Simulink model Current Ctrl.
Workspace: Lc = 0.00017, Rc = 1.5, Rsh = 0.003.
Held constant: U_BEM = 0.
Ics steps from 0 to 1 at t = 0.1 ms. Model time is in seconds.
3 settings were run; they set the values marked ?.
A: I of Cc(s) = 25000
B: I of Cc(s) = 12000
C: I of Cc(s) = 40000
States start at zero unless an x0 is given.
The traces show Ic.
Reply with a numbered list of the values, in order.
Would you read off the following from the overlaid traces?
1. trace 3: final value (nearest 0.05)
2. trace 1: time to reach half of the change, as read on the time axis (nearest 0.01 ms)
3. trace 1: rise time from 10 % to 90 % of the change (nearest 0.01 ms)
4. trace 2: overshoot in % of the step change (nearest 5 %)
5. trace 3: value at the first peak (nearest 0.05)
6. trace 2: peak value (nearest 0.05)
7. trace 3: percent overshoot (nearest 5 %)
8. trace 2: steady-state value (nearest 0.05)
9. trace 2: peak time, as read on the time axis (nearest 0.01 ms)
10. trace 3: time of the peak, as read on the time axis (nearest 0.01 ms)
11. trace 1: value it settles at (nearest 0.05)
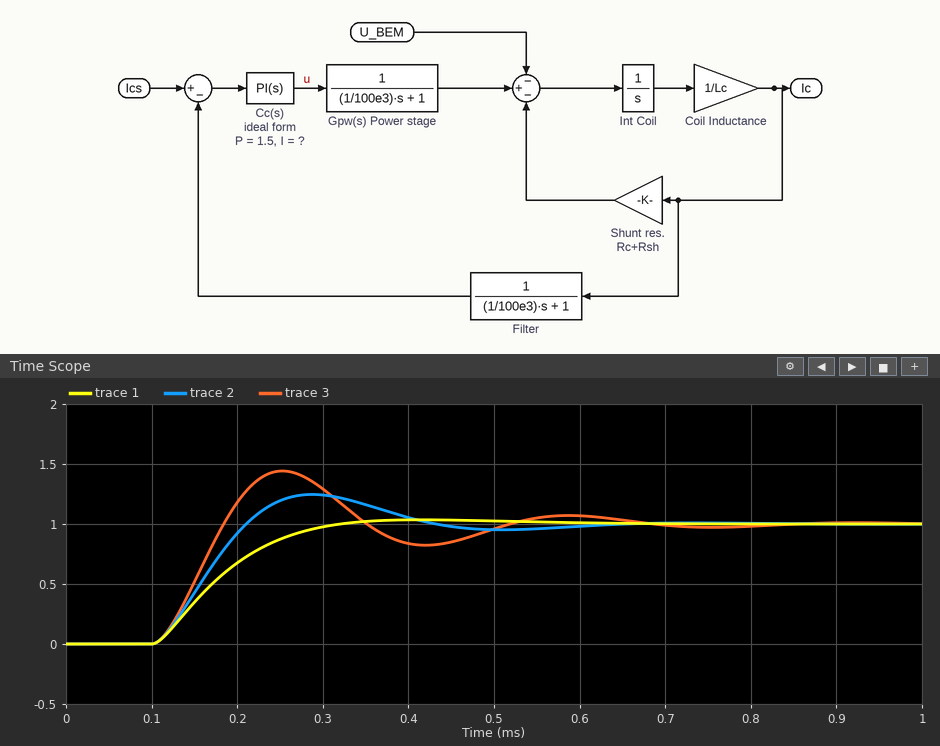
1. 1.00
2. 0.17 ms
3. 0.14 ms
4. 25 %
5. 1.45
6. 1.25
7. 45 %
8. 1.00
9. 0.29 ms
10. 0.25 ms
11. 1.00
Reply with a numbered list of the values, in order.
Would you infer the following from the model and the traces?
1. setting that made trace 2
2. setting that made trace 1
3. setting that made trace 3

1. A
2. B
3. C
